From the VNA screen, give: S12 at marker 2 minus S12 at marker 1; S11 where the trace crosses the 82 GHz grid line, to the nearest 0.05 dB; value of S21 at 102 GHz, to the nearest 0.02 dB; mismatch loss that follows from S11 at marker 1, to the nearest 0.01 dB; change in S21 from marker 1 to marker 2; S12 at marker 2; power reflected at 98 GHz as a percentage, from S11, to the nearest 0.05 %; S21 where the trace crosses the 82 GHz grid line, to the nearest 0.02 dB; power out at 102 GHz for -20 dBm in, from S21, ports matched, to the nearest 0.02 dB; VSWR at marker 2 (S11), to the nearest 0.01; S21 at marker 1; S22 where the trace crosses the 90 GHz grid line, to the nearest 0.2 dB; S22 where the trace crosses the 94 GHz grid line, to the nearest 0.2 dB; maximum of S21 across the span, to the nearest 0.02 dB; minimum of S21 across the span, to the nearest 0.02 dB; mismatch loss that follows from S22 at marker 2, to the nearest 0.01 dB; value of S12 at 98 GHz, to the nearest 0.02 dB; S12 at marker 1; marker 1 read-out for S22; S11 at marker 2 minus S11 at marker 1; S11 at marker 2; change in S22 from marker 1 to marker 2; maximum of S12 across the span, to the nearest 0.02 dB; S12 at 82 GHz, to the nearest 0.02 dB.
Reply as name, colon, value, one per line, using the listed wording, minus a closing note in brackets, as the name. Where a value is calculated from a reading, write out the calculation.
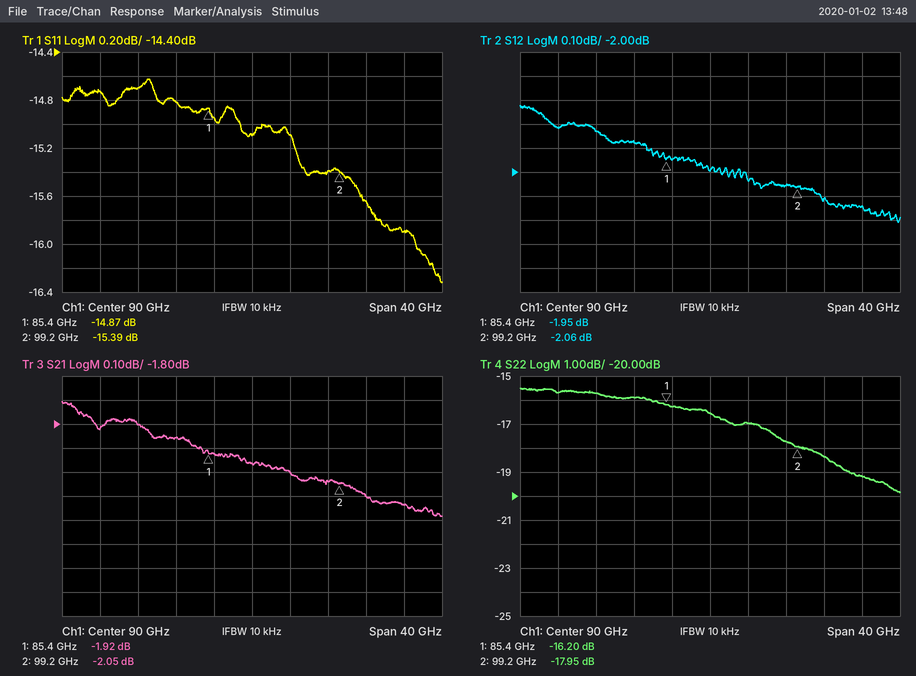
S12 at marker 2 minus S12 at marker 1: -2.06 − (-1.95) = -0.11 dB
S11 where the trace crosses the 82 GHz grid line, to the nearest 0.05 dB: -14.80 dB
value of S21 at 102 GHz, to the nearest 0.02 dB: -2.10 dB
mismatch loss that follows from S11 at marker 1, to the nearest 0.01 dB: −10 log10(1 − 10^(-14.87/10)) ≈ 0.14 dB
change in S21 from marker 1 to marker 2: -2.05 − (-1.92) = -0.13 dB
S12 at marker 2: -2.06 dB
power reflected at 98 GHz as a percentage, from S11, to the nearest 0.05 %: 10^(-15.4/10) ≈ 2.88 %, so 2.90 % to the nearest 0.05 %
S21 where the trace crosses the 82 GHz grid line, to the nearest 0.02 dB: -1.86 dB
power out at 102 GHz for -20 dBm in, from S21, ports matched, to the nearest 0.02 dB: -20 dBm + (-2.10 dB) = -22.10 dBm
VSWR at marker 2 (S11), to the nearest 0.01: (1 + 0.1700)/(1 − 0.1700) ≈ 1.41
S21 at marker 1: -1.92 dB
S22 where the trace crosses the 90 GHz grid line, to the nearest 0.2 dB: -16.6 dB
S22 where the trace crosses the 94 GHz grid line, to the nearest 0.2 dB: -17.0 dB
maximum of S21 across the span, to the nearest 0.02 dB: -1.70 dB
minimum of S21 across the span, to the nearest 0.02 dB: -2.18 dB
mismatch loss that follows from S22 at marker 2, to the nearest 0.01 dB: −10 log10(1 − 10^(-17.95/10)) ≈ 0.07 dB
value of S12 at 98 GHz, to the nearest 0.02 dB: -2.06 dB
S12 at marker 1: -1.95 dB
marker 1 read-out for S22: -16.20 dB
S11 at marker 2 minus S11 at marker 1: -15.39 − (-14.87) = -0.52 dB
S11 at marker 2: -15.39 dB
change in S22 from marker 1 to marker 2: -17.95 − (-16.2) = -1.75 dB
maximum of S12 across the span, to the nearest 0.02 dB: -1.72 dB
S12 at 82 GHz, to the nearest 0.02 dB: -1.88 dB
